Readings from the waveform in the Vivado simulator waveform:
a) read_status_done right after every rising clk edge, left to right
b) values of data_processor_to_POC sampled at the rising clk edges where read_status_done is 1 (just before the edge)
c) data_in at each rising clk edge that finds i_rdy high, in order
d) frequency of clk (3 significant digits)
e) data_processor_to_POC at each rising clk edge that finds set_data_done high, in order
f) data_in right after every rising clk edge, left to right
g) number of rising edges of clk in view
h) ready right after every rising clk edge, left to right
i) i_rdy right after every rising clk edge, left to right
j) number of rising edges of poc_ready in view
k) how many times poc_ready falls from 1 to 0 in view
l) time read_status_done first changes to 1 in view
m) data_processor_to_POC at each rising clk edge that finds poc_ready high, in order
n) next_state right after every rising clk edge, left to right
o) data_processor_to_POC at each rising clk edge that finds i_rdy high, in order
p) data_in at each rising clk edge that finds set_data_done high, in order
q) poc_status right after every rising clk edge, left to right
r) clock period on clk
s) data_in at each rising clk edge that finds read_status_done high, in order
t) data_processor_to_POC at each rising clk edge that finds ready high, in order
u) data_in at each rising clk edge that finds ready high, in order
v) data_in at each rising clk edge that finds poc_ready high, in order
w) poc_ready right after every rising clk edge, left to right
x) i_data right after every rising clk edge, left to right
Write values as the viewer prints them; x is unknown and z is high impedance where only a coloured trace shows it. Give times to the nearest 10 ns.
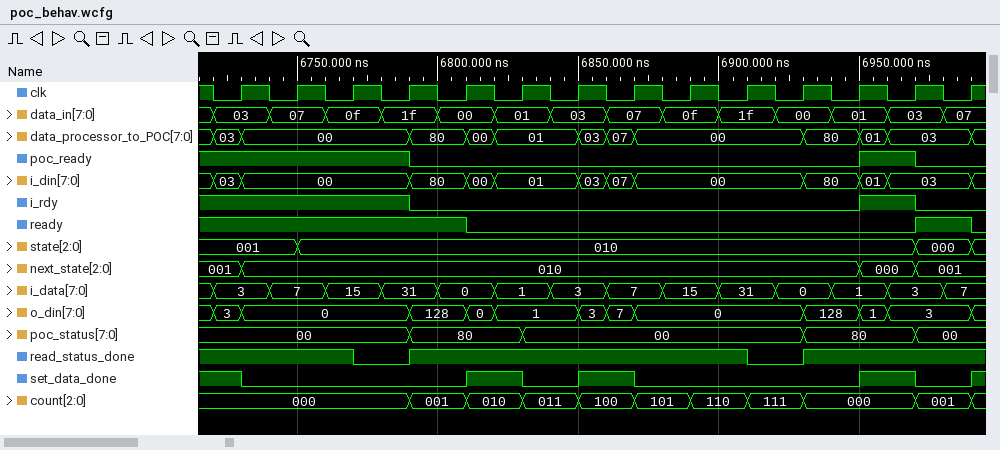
1 1 0 1 1 1 1 1 1 0 1 1 1 1
03, 00, 00, 80, 01, 01, 07, 00, 00, 80, 03, 03
03, 07, 0f, 1f, 03
50.0 MHz
03, 01, 07, 03
03, 07, 0f, 1f, 00, 01, 03, 07, 0f, 1f, 00, 01, 03, 07
14
1 1 1 1 0 0 0 0 0 0 0 0 1 0
1 1 1 0 0 0 0 0 0 0 0 1 0 0
1
2
6790 ns
03, 00, 00, 00, 03
010, 010, 010, 010, 010, 010, 010, 010, 010, 010, 010, 000, 001, 001
03, 00, 00, 00, 03
03, 01, 07, 03
00, 00, 00, 80, 80, 00, 00, 00, 00, 00, 80, 80, 00, 00
20 ns
03, 07, 0f, 00, 01, 03, 07, 0f, 1f, 01, 03, 07
03, 00, 00, 00, 80, 03
03, 07, 0f, 1f, 00, 07
03, 07, 0f, 1f, 03
1 1 1 0 0 0 0 0 0 0 0 1 0 0
3, 7, 15, 31, 0, 1, 3, 7, 15, 31, 0, 1, 3, 7
